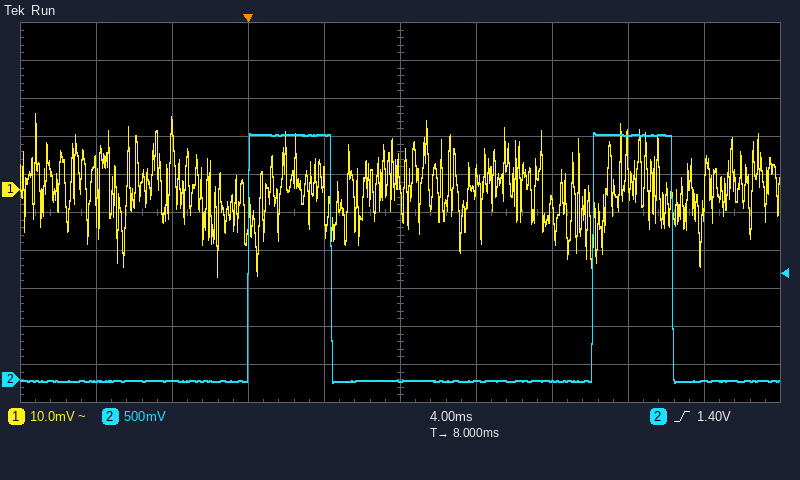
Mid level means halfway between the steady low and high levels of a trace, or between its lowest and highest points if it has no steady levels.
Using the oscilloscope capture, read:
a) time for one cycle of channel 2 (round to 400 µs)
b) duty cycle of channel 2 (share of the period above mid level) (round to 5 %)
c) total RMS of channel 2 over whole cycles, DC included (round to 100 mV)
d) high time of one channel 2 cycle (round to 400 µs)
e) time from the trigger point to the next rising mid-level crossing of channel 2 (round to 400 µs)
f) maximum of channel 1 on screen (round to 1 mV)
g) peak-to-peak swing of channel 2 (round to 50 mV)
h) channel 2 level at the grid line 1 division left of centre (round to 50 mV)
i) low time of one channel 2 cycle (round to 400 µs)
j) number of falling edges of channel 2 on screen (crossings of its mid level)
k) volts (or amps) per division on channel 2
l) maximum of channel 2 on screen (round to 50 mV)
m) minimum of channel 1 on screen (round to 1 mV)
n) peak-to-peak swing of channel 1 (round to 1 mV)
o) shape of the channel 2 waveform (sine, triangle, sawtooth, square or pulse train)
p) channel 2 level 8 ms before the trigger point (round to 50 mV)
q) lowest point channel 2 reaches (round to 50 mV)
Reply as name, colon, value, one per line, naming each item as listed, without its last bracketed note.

time for one cycle of channel 2: 18.0 ms
duty cycle of channel 2 (share of the period above mid level): 25 %
total RMS of channel 2 over whole cycles, DC included: 1.6 V
high time of one channel 2 cycle: 4.4 ms
time from the trigger point to the next rising mid-level crossing of channel 2: 18.0 ms
maximum of channel 1 on screen: 20 mV
peak-to-peak swing of channel 2: 3.30 V
channel 2 level at the grid line 1 division left of centre: 3.20 V
low time of one channel 2 cycle: 14.0 ms
number of falling edges of channel 2 on screen: 2
volts (or amps) per division on channel 2: 500 mV
maximum of channel 2 on screen: 3.25 V
minimum of channel 1 on screen: -23 mV
peak-to-peak swing of channel 1: 43 mV
shape of the channel 2 waveform: pulse train
channel 2 level 8 ms before the trigger point: 0 mV
lowest point channel 2 reaches: -50 mV
